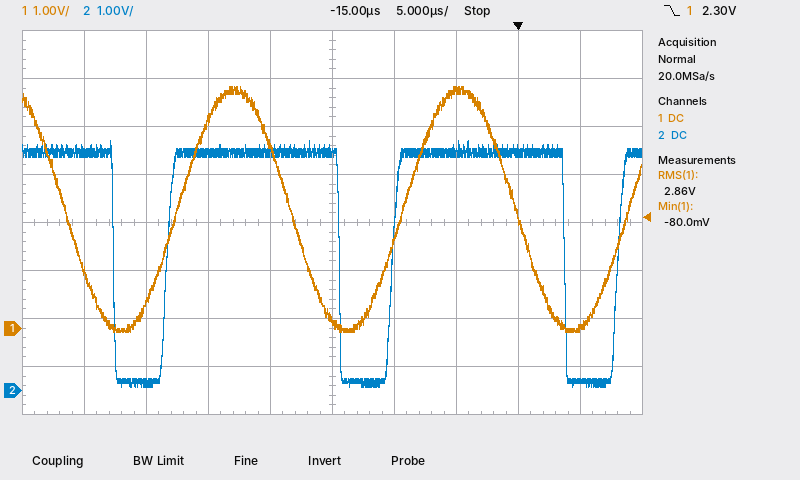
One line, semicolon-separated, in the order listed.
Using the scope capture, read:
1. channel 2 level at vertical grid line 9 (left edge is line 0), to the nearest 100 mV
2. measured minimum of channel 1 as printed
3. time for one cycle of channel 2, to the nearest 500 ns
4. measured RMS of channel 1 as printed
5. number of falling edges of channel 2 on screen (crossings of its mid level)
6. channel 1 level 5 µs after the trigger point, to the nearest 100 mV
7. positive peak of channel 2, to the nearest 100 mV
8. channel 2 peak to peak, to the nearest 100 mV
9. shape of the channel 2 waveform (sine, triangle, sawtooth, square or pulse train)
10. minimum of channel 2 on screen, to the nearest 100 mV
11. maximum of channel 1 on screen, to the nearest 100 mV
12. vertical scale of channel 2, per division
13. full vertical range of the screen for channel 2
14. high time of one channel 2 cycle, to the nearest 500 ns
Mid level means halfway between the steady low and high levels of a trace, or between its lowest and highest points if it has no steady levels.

200 mV; -80.0 mV; 18.0 µs; 2.86 V; 3; 0.0 V; 5.2 V; 5.1 V; pulse train; 100 mV; 5.0 V; 1 V; 8 V; 14.0 µs
